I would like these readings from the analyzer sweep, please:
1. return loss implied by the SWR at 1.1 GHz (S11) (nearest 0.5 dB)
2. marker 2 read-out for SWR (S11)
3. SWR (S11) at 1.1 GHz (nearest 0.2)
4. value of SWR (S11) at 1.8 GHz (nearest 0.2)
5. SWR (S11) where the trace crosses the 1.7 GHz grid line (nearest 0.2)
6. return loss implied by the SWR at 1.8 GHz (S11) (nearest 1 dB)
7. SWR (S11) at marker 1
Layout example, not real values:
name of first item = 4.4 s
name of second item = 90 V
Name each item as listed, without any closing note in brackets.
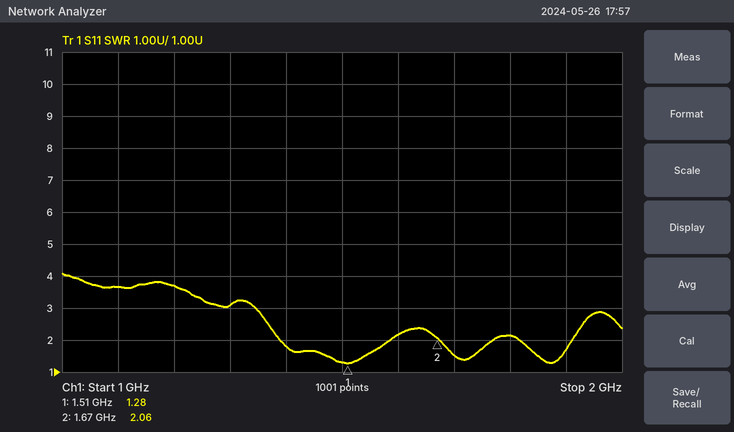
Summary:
return loss implied by the SWR at 1.1 GHz (S11) = 5.0 dB
marker 2 read-out for SWR = 2.06
SWR (S11) at 1.1 GHz = 3.6
value of SWR (S11) at 1.8 GHz = 2.2
SWR (S11) where the trace crosses the 1.7 GHz grid line = 1.6
return loss implied by the SWR at 1.8 GHz (S11) = 9 dB
SWR (S11) at marker 1 = 1.28
